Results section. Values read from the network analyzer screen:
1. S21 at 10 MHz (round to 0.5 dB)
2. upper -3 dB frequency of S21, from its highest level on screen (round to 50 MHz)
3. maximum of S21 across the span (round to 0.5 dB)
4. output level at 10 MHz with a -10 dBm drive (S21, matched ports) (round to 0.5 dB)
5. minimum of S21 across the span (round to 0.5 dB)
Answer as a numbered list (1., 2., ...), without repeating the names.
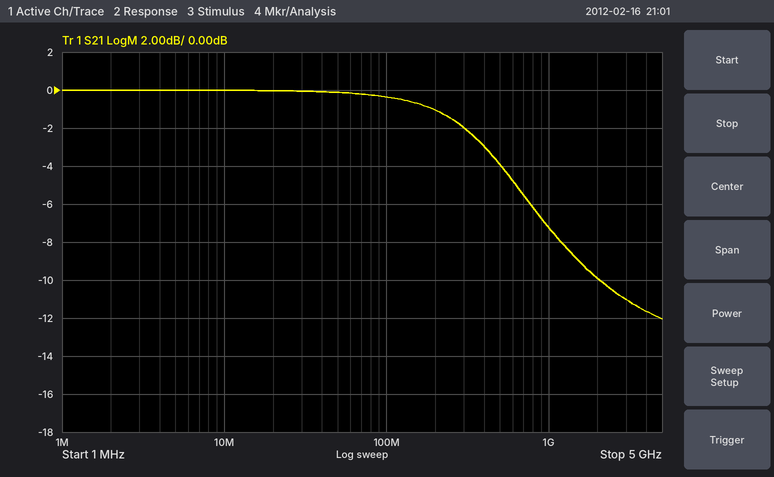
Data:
1. 0.0 dB
2. 400 MHz
3. 0.0 dB
4. -10.0 dBm
5. -12.0 dB
